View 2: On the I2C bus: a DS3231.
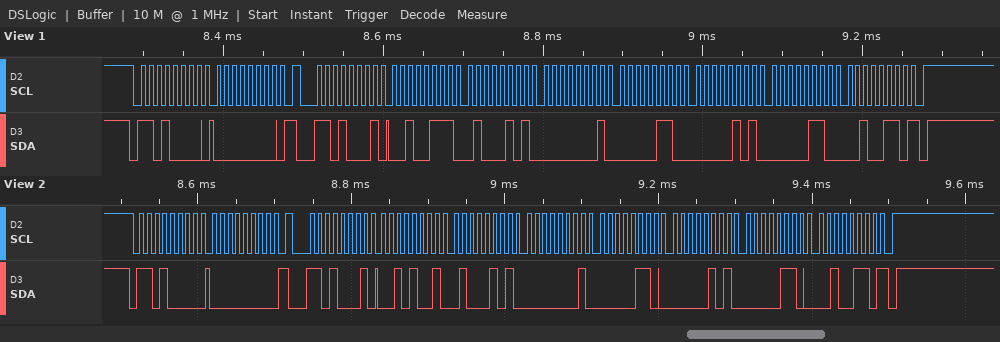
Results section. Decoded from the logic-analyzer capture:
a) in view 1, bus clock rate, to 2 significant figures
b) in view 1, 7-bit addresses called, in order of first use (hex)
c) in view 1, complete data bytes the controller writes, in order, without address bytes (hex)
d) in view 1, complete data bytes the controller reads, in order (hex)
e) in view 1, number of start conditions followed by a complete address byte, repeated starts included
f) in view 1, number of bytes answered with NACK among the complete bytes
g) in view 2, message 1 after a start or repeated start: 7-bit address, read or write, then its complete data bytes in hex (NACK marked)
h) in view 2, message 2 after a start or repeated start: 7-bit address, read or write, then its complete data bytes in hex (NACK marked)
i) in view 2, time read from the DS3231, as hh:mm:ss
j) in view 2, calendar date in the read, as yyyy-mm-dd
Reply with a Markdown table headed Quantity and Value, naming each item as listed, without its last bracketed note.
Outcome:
| Quantity | Value |
|---|---|
| in view 1, bus clock rate, to 2 significant figures | 100 kHz |
| in view 1, 7-bit addresses called, in order of first use | 0x68 |
| in view 1, complete data bytes the controller writes, in order, without address bytes | 00 |
| in view 1, complete data bytes the controller reads, in order | 27 45 01 06 05 06 26 |
| in view 1, number of start conditions followed by a complete address byte, repeated starts included | 2 |
| in view 1, number of bytes answered with NACK among the complete bytes | 1 |
| in view 2, message 1 after a start or repeated start: 7-bit address, read or write, then its complete data bytes in hex | 0x68 write: 00 |
| in view 2, message 2 after a start or repeated start: 7-bit address, read or write, then its complete data bytes in hex | 0x68 read: 29 45 01 06 05 06 26 NACK |
| in view 2, time read from the DS3231, as hh:mm:ss | 01:45:29 |
| in view 2, calendar date in the read, as yyyy-mm-dd | 2026-06-05 |
